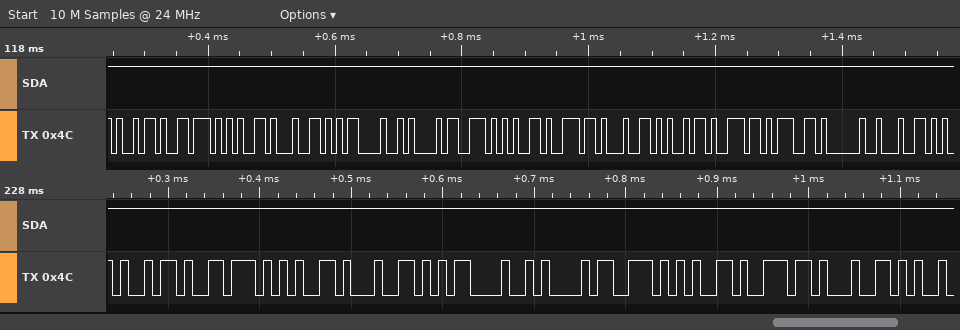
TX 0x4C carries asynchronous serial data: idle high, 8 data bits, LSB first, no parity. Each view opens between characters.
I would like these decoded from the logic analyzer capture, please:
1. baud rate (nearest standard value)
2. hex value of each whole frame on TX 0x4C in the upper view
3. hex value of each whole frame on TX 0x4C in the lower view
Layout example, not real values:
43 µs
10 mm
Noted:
115200 baud
69, 76, 65, 64, 0D, 0A, 73, 65, 6E, 64, 69, 6E, 67, 20, 64
69, 76, 65, 64, 0D, 0A, 73, 65, 6E, 64
